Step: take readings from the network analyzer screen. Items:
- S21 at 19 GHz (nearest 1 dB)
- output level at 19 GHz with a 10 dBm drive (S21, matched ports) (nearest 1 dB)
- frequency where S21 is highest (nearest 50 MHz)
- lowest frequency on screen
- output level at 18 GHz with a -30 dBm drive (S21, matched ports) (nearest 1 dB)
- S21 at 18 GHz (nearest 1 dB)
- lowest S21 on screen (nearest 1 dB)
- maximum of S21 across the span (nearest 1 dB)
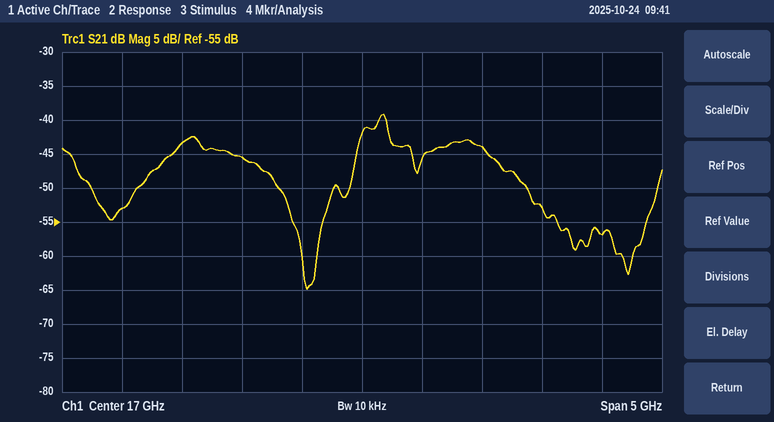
-57 dB
-47 dBm
17.20 GHz
14.5 GHz
-74 dBm
-44 dB
-65 dB
-39 dB
